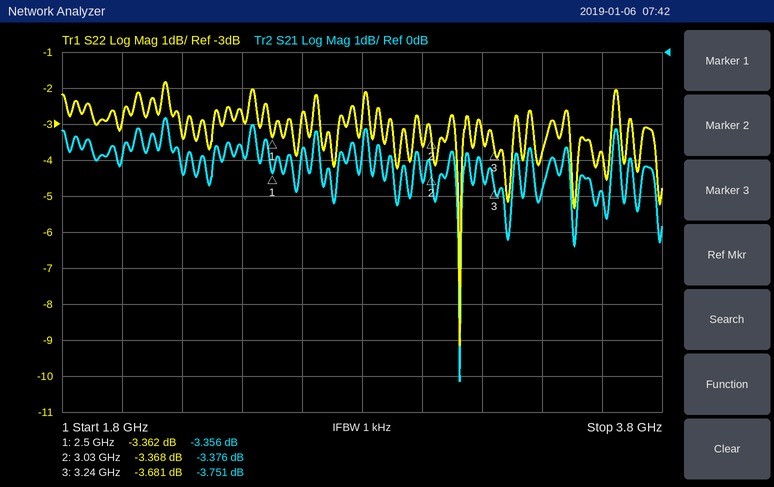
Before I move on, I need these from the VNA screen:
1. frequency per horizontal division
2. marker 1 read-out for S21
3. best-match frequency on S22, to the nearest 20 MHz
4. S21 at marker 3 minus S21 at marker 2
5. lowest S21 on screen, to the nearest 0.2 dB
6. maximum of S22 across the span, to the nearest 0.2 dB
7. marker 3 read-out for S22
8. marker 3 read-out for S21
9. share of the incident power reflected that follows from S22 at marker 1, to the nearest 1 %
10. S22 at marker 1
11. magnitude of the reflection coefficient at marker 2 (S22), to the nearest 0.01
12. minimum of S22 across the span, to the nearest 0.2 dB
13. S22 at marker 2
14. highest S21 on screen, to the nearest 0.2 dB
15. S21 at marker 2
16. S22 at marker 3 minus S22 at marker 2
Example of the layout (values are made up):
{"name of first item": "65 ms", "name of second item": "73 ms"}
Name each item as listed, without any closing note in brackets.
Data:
{"frequency per horizontal division": "200 MHz", "marker 1 read-out for S21": "-3.356 dB", "best-match frequency on S22, to the nearest 20 MHz": "3.12 GHz", "S21 at marker 3 minus S21 at marker 2": "-0.375 dB", "lowest S21 on screen, to the nearest 0.2 dB": "-9.2 dB", "maximum of S22 across the span, to the nearest 0.2 dB": "-1.8 dB", "marker 3 read-out for S22": "-3.681 dB", "marker 3 read-out for S21": "-3.751 dB", "share of the incident power reflected that follows from S22 at marker 1, to the nearest 1 %": "46 %", "S22 at marker 1": "-3.362 dB", "magnitude of the reflection coefficient at marker 2 (S22), to the nearest 0.01": "0.68", "minimum of S22 across the span, to the nearest 0.2 dB": "-9.2 dB", "S22 at marker 2": "-3.368 dB", "highest S21 on screen, to the nearest 0.2 dB": "-1.8 dB", "S21 at marker 2": "-3.376 dB", "S22 at marker 3 minus S22 at marker 2": "-0.313 dB"}
